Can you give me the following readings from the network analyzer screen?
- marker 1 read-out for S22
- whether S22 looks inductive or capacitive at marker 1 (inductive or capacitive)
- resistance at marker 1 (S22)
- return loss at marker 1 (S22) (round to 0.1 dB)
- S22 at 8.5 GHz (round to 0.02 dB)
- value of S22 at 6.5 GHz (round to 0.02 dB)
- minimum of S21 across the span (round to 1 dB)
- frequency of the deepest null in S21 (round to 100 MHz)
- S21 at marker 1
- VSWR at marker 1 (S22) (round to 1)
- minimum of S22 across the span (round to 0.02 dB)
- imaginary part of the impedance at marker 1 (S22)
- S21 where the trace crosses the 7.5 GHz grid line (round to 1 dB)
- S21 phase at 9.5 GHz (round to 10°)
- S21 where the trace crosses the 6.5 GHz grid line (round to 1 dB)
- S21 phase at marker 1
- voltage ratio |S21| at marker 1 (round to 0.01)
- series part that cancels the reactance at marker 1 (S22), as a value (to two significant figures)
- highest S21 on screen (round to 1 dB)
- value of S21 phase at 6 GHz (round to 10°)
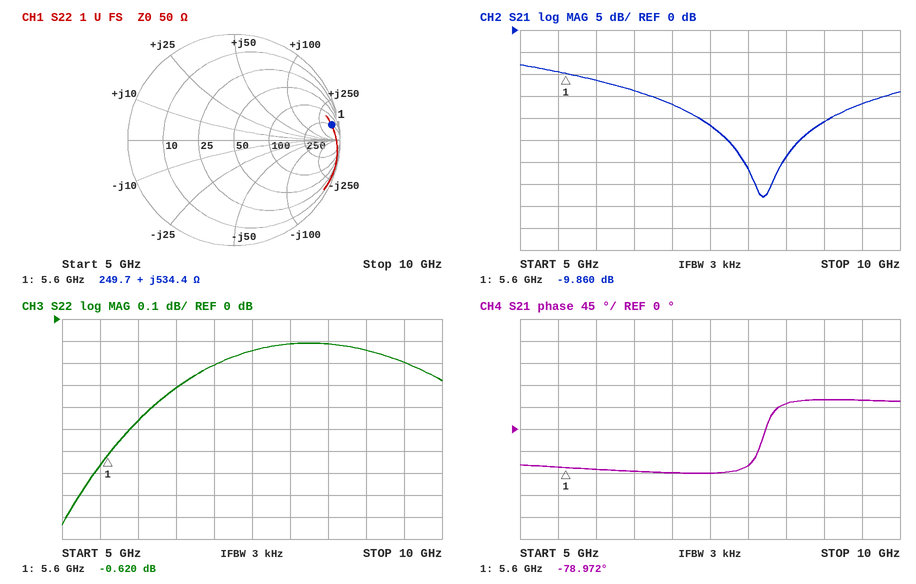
-0.620 dB
inductive
249.7 Ω
0.6 dB
-0.12 dB
-0.32 dB
-38 dB
8.2 GHz
-9.860 dB
28
-0.94 dB
+534.4 Ω
-22 dB
60°
-14 dB
-78.972°
0.32
53 fF
-8 dB
-80°
